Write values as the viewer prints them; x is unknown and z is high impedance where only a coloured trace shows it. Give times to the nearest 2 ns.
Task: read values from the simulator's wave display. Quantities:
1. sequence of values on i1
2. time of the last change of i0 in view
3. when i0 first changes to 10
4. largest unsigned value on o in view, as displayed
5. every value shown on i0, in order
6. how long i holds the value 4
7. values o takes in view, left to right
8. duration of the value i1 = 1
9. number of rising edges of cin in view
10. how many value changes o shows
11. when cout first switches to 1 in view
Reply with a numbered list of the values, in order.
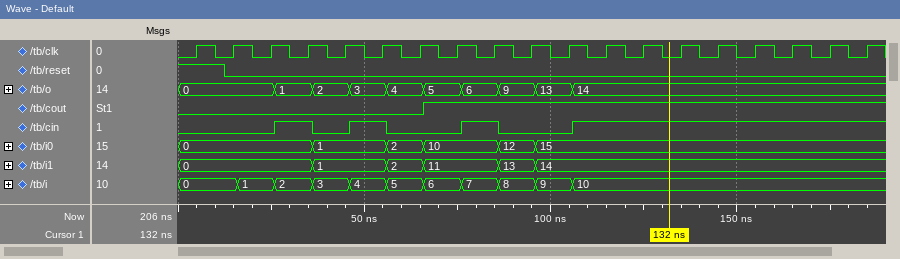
1. 0, 1, 2, 11, 13, 14
2. 96 ns
3. 66 ns
4. 14
5. 0, 1, 2, 10, 12, 15
6. 10 ns
7. 0, 1, 2, 3, 4, 5, 6, 9, 13, 14
8. 20 ns
9. 4
10. 9
11. 66 ns
